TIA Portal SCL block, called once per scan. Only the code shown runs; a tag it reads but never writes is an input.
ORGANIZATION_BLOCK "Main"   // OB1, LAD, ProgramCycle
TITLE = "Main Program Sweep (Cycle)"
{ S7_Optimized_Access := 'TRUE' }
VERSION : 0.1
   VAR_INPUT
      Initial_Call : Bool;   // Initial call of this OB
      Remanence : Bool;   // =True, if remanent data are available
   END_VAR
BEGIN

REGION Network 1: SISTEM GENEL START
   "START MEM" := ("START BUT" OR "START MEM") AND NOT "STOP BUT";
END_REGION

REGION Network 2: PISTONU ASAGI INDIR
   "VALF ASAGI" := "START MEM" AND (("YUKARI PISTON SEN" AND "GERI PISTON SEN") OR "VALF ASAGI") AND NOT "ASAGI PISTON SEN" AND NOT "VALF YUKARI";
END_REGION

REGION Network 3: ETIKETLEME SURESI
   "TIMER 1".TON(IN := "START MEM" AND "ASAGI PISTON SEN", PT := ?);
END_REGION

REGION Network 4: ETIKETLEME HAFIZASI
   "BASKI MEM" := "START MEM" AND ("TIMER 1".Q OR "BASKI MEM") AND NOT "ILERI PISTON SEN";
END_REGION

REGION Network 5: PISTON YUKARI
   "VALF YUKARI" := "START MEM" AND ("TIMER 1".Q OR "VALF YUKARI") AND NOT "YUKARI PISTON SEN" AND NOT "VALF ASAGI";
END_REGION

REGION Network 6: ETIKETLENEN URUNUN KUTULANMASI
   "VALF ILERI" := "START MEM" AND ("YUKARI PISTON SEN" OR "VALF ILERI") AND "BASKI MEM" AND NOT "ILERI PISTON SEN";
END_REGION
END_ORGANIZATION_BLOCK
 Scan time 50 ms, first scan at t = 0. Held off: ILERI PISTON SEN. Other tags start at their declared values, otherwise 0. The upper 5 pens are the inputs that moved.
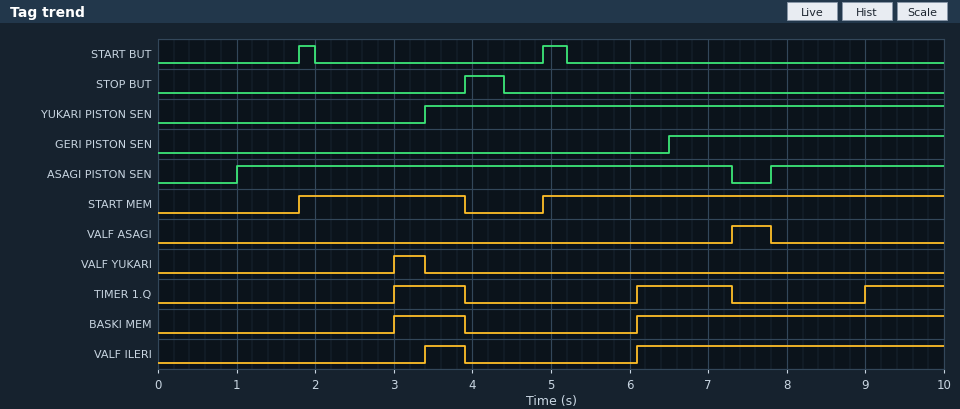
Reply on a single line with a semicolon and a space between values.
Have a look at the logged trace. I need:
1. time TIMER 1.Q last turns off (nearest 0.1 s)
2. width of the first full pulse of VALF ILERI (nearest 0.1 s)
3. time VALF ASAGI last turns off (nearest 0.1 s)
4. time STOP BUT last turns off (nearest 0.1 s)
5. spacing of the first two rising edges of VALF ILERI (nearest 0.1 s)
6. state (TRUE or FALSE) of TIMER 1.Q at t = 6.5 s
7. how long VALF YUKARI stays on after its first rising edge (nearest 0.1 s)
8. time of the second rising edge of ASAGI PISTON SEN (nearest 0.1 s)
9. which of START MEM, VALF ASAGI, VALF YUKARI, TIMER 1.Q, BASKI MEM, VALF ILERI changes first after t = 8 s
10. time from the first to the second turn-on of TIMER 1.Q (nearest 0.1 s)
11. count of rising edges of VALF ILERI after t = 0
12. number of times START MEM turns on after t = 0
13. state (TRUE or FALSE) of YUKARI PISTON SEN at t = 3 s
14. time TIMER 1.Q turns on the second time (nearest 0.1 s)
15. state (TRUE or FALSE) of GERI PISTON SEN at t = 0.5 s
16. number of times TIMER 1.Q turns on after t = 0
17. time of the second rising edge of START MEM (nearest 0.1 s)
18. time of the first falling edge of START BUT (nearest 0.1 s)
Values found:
7.3 s; 0.5 s; 7.8 s; 4.4 s; 2.7 s; TRUE; 0.4 s; 7.8 s; TIMER 1.Q; 3.1 s; 2; 2; FALSE; 6.1 s; FALSE; 3; 4.9 s; 2.0 s
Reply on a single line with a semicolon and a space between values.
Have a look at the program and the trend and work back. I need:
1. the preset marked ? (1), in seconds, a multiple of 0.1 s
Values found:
1.2 s
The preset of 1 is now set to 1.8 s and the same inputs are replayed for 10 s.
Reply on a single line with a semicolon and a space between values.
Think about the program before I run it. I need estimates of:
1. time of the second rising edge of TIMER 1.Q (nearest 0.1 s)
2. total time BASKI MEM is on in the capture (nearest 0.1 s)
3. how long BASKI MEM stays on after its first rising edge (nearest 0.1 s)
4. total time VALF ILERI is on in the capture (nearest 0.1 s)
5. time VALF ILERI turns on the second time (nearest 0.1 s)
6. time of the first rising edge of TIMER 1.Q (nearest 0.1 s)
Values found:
6.7 s; 3.6 s; 0.3 s; 3.6 s; 6.7 s; 3.6 s
